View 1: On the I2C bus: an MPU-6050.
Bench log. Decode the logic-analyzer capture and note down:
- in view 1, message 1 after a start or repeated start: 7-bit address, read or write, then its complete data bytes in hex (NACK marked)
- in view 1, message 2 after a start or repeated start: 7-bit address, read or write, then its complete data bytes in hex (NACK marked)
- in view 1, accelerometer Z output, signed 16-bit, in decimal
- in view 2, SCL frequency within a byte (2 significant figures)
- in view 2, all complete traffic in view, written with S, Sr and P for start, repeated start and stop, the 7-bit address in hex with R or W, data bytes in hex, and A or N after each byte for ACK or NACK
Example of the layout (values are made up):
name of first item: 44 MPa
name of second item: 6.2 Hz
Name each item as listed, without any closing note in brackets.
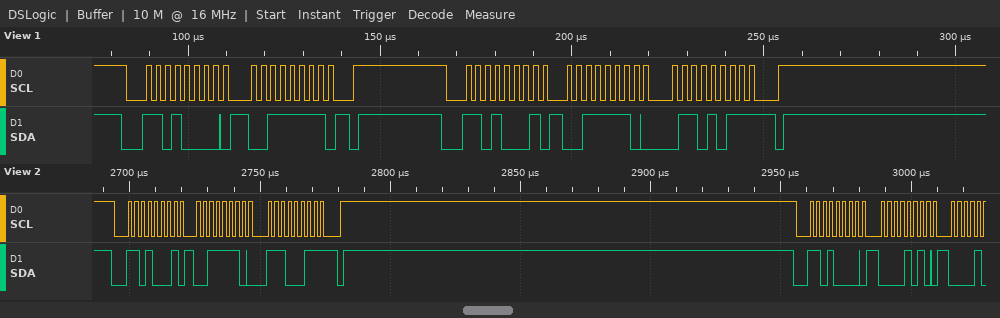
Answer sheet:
in view 1, message 1 after a start or repeated start: 7-bit address, read or write, then its complete data bytes in hex: 0x68 write: 3F
in view 1, message 2 after a start or repeated start: 7-bit address, read or write, then its complete data bytes in hex: 0x68 read: 3E 6B NACK
in view 1, accelerometer Z output, signed 16-bit, in decimal: 15979
in view 2, SCL frequency within a byte: 400 kHz
in view 2, all complete traffic in view, written with S, Sr and P for start, repeated start and stop, the 7-bit address in hex with R or W, data bytes in hex, and A or N after each byte for ACK or NACK: S 68R A 3E A E3 N P S 68W A 0A A
